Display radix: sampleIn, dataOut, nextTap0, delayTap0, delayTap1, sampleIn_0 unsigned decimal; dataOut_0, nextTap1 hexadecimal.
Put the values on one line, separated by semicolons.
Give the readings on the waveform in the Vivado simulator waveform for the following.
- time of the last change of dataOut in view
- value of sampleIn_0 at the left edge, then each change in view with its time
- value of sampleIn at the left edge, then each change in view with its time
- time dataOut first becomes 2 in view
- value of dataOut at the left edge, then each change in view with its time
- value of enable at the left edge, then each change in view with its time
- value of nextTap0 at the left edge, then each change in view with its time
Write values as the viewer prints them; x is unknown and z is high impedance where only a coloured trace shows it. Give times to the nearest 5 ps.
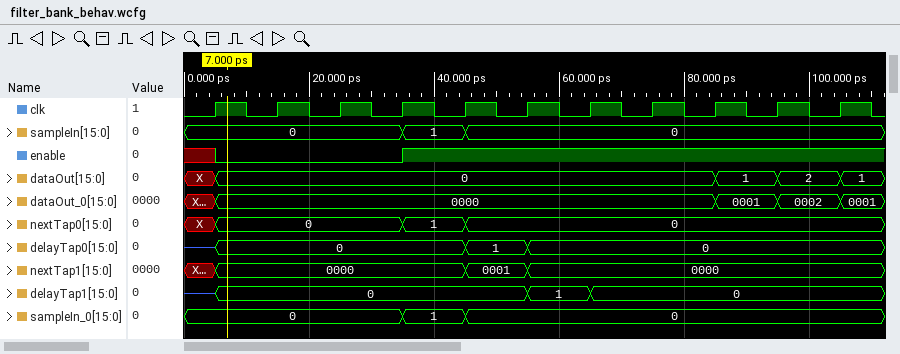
105 ps; 0, 1 at 35 ps, 0 at 45 ps; 0, 1 at 35 ps, 0 at 45 ps; 95 ps; X, 0 at 5 ps, 1 at 85 ps, 2 at 95 ps, 1 at 105 ps; x, 0 at 5 ps, 1 at 35 ps; X, 0 at 5 ps, 1 at 35 ps, 0 at 45 ps
